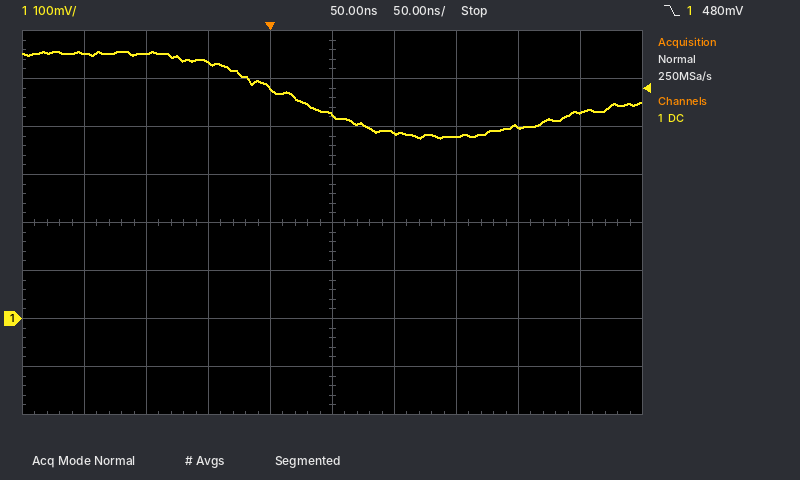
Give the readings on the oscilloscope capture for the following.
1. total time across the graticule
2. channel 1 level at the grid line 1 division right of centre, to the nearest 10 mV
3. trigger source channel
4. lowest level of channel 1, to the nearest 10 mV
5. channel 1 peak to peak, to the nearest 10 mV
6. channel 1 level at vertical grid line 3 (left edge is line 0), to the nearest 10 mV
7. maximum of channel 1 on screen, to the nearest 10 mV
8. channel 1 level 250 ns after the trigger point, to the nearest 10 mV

500 ns
390 mV
channel 1
380 mV
180 mV
530 mV
560 mV
430 mV
